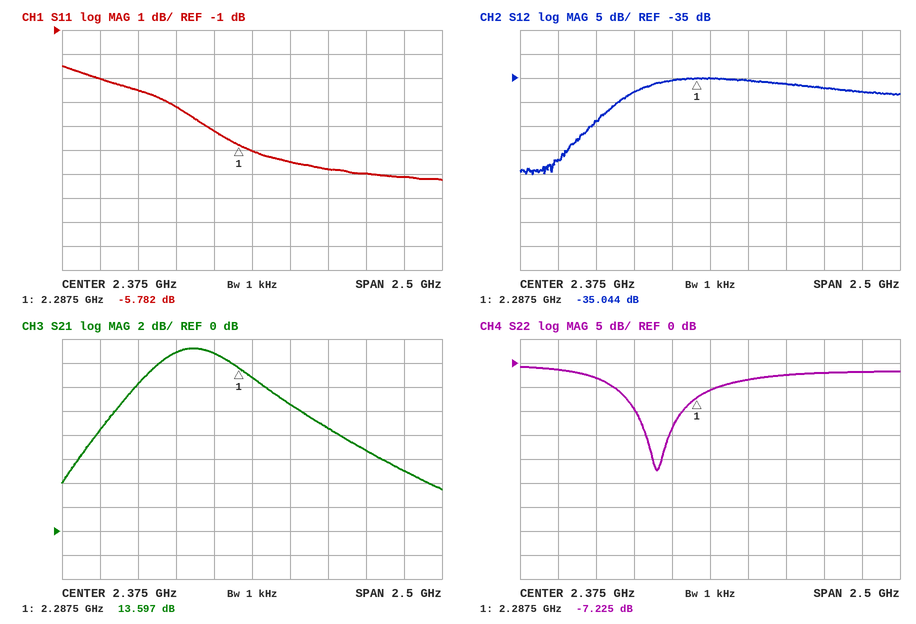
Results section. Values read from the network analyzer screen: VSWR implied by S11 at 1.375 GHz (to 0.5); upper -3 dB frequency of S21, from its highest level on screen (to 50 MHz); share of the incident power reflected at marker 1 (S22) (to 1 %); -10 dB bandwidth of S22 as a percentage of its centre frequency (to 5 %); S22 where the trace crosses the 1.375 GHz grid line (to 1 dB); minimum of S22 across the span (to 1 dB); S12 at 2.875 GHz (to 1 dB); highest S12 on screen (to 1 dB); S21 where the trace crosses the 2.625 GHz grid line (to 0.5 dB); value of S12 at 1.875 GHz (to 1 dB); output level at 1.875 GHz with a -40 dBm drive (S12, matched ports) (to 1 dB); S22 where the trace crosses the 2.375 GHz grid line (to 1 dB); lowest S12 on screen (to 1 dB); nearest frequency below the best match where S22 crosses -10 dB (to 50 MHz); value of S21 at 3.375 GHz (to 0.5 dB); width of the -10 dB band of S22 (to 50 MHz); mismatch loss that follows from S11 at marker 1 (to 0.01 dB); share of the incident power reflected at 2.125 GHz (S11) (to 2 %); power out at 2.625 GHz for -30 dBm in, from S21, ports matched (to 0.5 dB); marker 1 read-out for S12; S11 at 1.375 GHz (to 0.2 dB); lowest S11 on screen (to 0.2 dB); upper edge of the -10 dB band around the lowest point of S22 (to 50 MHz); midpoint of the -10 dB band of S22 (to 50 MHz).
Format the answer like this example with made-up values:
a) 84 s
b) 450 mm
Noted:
a) 6.0
b) 2.45 GHz
c) 19 %
d) 15 %
e) -1 dB
f) -22 dB
g) -36 dB
h) -35 dB
i) 10.5 dB
j) -38 dB
k) -78 dBm
l) -6 dB
m) -55 dB
n) 1.90 GHz
o) 5.0 dB
p) 300 MHz
q) 1.33 dB
r) 30 %
s) -19.5 dBm
t) -35.044 dB
u) -3.0 dB
v) -7.2 dB
w) 2.20 GHz
x) 2.05 GHz
